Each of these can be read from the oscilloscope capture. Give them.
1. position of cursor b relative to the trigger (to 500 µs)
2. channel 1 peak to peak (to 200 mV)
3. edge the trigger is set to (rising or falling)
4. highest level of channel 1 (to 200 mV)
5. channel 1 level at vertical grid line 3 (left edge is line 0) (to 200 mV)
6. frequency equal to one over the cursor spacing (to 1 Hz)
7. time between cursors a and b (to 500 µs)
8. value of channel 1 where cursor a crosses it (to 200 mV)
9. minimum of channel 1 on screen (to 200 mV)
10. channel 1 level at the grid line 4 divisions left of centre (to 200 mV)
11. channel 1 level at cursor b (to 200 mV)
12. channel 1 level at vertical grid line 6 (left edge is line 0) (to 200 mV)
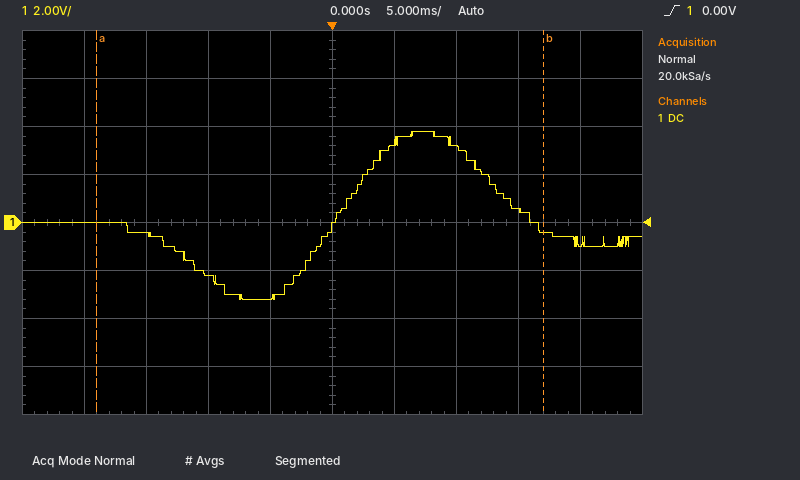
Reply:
+17.0 ms
7.0 V
rising
3.8 V
-2.2 V
28 Hz
36.0 ms
0.0 V
-3.2 V
0.0 V
-400 mV
3.4 V
